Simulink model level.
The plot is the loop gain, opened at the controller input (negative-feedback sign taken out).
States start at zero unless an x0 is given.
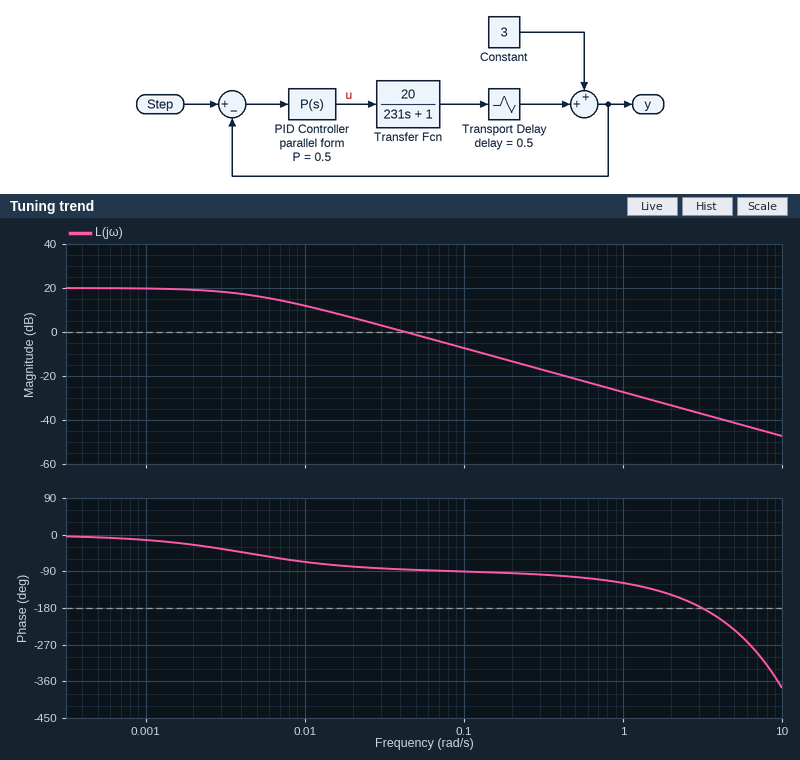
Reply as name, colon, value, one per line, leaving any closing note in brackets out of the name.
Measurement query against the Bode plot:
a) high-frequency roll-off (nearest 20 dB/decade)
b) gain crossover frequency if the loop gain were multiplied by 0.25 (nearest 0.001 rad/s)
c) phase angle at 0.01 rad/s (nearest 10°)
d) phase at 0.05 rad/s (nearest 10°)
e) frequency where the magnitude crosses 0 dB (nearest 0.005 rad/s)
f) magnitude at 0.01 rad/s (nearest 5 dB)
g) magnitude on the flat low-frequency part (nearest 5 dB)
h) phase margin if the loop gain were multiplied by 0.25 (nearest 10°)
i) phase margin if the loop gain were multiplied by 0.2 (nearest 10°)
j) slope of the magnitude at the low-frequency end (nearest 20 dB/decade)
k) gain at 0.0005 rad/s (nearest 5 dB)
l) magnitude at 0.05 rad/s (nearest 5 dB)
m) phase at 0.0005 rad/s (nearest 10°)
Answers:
high-frequency roll-off: -20 dB/decade
gain crossover frequency if the loop gain were multiplied by 0.25: 0.010 rad/s
phase angle at 0.01 rad/s: -70°
phase at 0.05 rad/s: -90°
frequency where the magnitude crosses 0 dB: 0.045 rad/s
magnitude at 0.01 rad/s: 10 dB
magnitude on the flat low-frequency part: 20 dB
phase margin if the loop gain were multiplied by 0.25: 110°
phase margin if the loop gain were multiplied by 0.2: 120°
slope of the magnitude at the low-frequency end: 0 dB/decade
gain at 0.0005 rad/s: 20 dB
magnitude at 0.05 rad/s: 0 dB
phase at 0.0005 rad/s: -10°
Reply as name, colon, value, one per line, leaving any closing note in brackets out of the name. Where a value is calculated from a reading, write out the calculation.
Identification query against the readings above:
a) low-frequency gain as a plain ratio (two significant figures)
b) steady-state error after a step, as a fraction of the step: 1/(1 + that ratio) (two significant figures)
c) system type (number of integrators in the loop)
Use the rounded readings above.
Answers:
low-frequency gain as a plain ratio: 10^(20 / 20) = 10
steady-state error after a step, as a fraction of the step: 1/(1 + that ratio): 1 / (1 + 10) = 0.091
system type: 0
